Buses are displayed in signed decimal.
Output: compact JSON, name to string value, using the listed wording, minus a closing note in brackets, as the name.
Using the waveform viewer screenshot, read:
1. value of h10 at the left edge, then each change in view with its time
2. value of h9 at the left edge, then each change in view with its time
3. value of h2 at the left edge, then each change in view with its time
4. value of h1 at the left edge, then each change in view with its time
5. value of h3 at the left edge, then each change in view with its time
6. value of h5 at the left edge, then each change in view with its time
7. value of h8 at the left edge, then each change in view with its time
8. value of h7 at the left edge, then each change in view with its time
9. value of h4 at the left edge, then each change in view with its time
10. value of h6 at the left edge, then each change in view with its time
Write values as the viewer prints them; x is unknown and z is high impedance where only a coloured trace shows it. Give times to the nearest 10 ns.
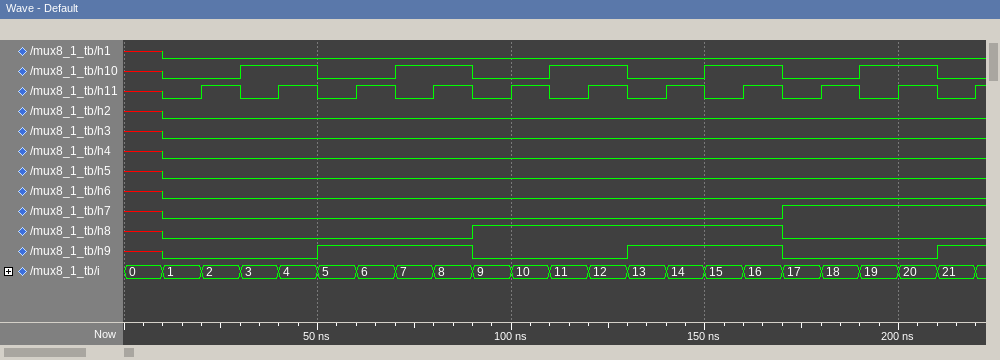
{"value of h10 at the left edge, then each change in view with its time": "x, 0 at 10 ns, 1 at 30 ns, 0 at 50 ns, 1 at 70 ns, 0 at 90 ns, 1 at 110 ns, 0 at 130 ns, 1 at 150 ns, 0 at 170 ns, 1 at 190 ns, 0 at 210 ns", "value of h9 at the left edge, then each change in view with its time": "x, 0 at 10 ns, 1 at 50 ns, 0 at 90 ns, 1 at 130 ns, 0 at 170 ns, 1 at 210 ns", "value of h2 at the left edge, then each change in view with its time": "x, 0 at 10 ns", "value of h1 at the left edge, then each change in view with its time": "x, 0 at 10 ns", "value of h3 at the left edge, then each change in view with its time": "x, 0 at 10 ns", "value of h5 at the left edge, then each change in view with its time": "x, 0 at 10 ns", "value of h8 at the left edge, then each change in view with its time": "x, 0 at 10 ns, 1 at 90 ns, 0 at 170 ns", "value of h7 at the left edge, then each change in view with its time": "x, 0 at 10 ns, 1 at 170 ns", "value of h4 at the left edge, then each change in view with its time": "x, 0 at 10 ns", "value of h6 at the left edge, then each change in view with its time": "x, 0 at 10 ns"}
